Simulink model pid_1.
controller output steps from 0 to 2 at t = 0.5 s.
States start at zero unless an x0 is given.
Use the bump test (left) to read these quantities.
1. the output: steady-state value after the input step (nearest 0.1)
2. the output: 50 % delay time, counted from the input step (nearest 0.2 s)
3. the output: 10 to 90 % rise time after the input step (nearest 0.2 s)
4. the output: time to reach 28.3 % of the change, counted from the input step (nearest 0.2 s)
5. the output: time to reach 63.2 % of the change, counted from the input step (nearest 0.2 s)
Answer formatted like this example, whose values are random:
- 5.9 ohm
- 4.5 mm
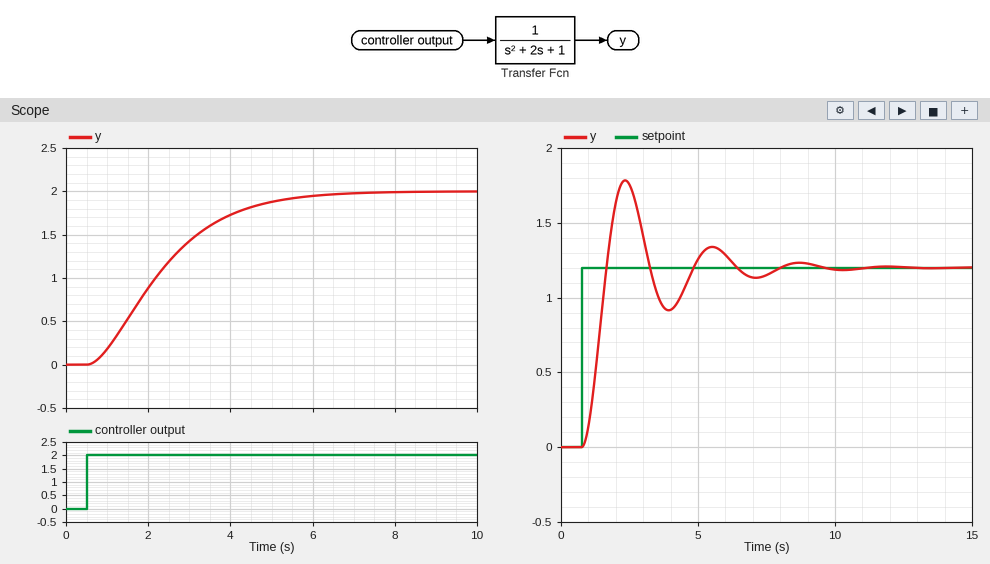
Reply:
- 2.0
- 1.6 s
- 3.4 s
- 1.0 s
- 2.2 s
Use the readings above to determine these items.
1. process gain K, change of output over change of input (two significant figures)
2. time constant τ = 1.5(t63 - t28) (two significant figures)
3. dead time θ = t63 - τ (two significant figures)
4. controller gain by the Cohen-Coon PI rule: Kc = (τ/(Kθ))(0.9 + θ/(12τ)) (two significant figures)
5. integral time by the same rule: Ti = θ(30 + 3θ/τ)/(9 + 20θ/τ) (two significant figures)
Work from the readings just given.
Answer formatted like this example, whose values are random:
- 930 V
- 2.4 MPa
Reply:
- 1.0
- 1.8 s
- 0.40 s
- 4.1
- 0.91 s
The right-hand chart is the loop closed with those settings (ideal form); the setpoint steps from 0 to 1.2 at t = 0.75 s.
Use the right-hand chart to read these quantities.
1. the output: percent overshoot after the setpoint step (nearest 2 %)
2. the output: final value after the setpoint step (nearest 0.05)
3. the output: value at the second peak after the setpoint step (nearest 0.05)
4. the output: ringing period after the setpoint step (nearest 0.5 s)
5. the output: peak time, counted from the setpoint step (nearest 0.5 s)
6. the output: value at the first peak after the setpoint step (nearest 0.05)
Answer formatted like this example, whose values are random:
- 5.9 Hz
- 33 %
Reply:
- 48 %
- 1.20
- 1.35
- 3.0 s
- 1.5 s
- 1.80
